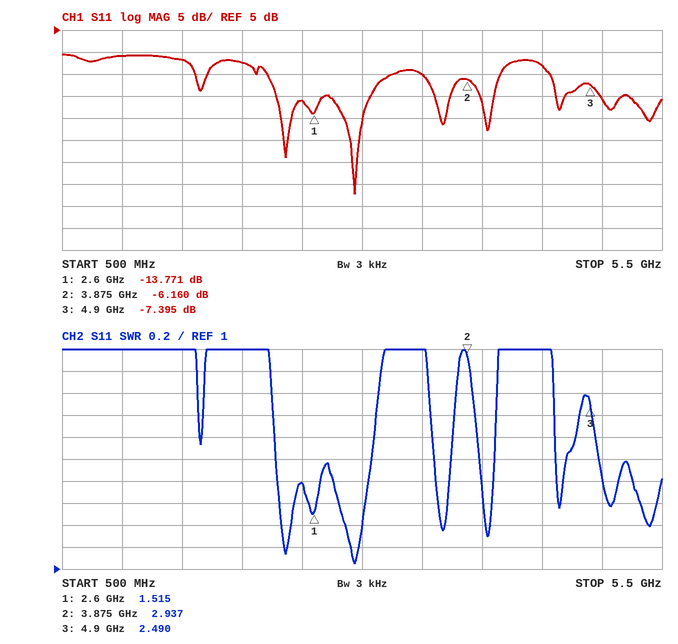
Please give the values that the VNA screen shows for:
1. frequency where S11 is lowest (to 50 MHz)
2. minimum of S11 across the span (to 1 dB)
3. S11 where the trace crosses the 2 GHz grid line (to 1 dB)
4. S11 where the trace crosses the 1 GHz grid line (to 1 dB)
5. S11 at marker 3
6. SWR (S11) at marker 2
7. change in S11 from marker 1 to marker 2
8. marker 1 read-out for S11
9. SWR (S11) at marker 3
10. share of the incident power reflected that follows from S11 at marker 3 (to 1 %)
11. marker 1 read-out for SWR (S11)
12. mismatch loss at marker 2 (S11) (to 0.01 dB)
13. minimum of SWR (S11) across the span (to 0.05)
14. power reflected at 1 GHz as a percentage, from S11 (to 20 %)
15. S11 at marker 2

2.95 GHz
-32 dB
-2 dB
-1 dB
-7.395 dB
2.937
7.611 dB
-13.771 dB
2.490
18 %
1.515
1.20 dB
1.05
80 %
-6.160 dB
